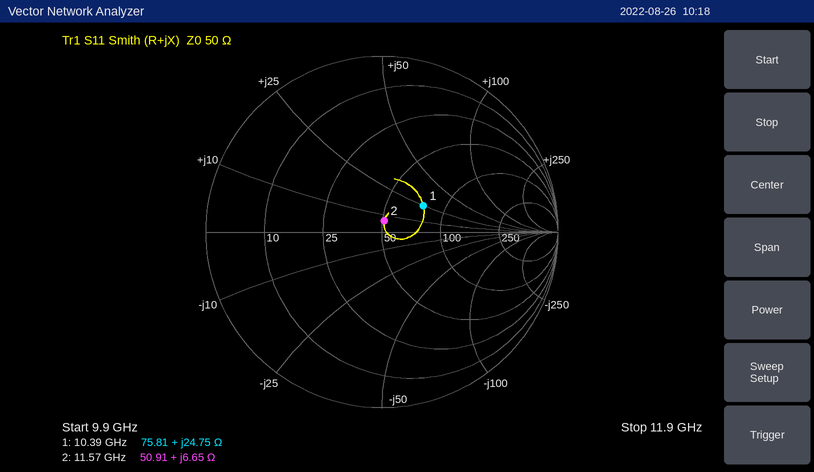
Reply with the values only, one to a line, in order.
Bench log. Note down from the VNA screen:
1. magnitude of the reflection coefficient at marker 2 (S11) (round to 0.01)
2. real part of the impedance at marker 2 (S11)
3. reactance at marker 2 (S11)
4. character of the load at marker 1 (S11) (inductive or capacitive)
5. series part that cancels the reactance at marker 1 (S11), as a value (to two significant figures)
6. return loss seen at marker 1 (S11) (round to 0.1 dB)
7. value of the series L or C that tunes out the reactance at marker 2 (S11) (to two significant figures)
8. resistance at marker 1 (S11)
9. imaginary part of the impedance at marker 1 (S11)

0.07
50.91 Ω
+6.65 Ω
inductive
620 fF
11.1 dB
2.1 pF
75.81 Ω
+24.75 Ω
